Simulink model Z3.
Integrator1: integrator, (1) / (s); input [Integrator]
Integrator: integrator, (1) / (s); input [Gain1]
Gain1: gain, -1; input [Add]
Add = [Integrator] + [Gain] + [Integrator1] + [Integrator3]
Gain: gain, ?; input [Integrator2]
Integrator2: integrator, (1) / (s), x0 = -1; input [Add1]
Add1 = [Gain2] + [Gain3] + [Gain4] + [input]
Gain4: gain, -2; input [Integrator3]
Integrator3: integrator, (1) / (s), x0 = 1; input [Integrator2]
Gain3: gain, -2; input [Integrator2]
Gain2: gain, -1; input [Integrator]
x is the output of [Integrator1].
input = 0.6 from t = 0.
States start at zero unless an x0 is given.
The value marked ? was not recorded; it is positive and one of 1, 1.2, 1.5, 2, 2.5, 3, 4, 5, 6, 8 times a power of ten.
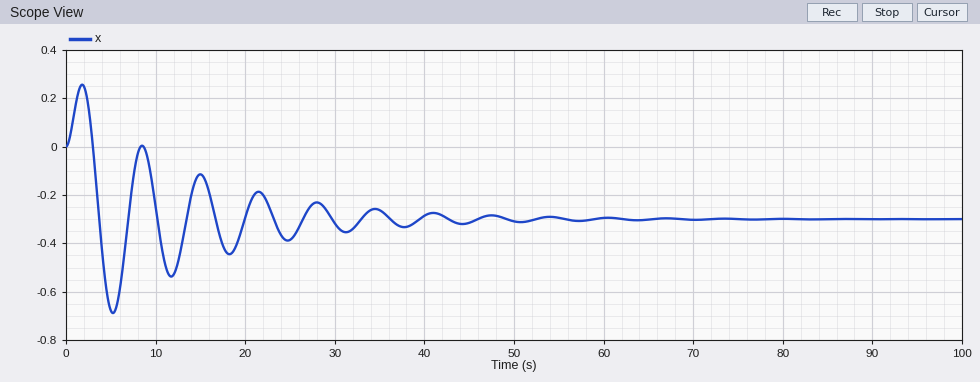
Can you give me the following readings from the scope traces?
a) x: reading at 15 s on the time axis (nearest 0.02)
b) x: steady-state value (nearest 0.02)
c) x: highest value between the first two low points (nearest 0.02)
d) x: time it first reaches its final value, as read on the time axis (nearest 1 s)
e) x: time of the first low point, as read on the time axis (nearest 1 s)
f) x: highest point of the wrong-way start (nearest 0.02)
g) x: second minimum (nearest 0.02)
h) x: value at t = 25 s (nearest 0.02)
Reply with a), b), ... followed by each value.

a) -0.12
b) -0.30
c) 0.00
d) 4 s
e) 5 s
f) 0.26
g) -0.54
h) -0.38
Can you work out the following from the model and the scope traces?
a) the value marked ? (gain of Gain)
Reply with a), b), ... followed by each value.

a) 1.5
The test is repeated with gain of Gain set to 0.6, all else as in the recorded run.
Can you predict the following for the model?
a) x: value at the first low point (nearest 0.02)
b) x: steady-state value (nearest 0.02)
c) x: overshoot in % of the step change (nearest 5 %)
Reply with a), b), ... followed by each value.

a) -0.36
b) -0.30
c) 20 %
